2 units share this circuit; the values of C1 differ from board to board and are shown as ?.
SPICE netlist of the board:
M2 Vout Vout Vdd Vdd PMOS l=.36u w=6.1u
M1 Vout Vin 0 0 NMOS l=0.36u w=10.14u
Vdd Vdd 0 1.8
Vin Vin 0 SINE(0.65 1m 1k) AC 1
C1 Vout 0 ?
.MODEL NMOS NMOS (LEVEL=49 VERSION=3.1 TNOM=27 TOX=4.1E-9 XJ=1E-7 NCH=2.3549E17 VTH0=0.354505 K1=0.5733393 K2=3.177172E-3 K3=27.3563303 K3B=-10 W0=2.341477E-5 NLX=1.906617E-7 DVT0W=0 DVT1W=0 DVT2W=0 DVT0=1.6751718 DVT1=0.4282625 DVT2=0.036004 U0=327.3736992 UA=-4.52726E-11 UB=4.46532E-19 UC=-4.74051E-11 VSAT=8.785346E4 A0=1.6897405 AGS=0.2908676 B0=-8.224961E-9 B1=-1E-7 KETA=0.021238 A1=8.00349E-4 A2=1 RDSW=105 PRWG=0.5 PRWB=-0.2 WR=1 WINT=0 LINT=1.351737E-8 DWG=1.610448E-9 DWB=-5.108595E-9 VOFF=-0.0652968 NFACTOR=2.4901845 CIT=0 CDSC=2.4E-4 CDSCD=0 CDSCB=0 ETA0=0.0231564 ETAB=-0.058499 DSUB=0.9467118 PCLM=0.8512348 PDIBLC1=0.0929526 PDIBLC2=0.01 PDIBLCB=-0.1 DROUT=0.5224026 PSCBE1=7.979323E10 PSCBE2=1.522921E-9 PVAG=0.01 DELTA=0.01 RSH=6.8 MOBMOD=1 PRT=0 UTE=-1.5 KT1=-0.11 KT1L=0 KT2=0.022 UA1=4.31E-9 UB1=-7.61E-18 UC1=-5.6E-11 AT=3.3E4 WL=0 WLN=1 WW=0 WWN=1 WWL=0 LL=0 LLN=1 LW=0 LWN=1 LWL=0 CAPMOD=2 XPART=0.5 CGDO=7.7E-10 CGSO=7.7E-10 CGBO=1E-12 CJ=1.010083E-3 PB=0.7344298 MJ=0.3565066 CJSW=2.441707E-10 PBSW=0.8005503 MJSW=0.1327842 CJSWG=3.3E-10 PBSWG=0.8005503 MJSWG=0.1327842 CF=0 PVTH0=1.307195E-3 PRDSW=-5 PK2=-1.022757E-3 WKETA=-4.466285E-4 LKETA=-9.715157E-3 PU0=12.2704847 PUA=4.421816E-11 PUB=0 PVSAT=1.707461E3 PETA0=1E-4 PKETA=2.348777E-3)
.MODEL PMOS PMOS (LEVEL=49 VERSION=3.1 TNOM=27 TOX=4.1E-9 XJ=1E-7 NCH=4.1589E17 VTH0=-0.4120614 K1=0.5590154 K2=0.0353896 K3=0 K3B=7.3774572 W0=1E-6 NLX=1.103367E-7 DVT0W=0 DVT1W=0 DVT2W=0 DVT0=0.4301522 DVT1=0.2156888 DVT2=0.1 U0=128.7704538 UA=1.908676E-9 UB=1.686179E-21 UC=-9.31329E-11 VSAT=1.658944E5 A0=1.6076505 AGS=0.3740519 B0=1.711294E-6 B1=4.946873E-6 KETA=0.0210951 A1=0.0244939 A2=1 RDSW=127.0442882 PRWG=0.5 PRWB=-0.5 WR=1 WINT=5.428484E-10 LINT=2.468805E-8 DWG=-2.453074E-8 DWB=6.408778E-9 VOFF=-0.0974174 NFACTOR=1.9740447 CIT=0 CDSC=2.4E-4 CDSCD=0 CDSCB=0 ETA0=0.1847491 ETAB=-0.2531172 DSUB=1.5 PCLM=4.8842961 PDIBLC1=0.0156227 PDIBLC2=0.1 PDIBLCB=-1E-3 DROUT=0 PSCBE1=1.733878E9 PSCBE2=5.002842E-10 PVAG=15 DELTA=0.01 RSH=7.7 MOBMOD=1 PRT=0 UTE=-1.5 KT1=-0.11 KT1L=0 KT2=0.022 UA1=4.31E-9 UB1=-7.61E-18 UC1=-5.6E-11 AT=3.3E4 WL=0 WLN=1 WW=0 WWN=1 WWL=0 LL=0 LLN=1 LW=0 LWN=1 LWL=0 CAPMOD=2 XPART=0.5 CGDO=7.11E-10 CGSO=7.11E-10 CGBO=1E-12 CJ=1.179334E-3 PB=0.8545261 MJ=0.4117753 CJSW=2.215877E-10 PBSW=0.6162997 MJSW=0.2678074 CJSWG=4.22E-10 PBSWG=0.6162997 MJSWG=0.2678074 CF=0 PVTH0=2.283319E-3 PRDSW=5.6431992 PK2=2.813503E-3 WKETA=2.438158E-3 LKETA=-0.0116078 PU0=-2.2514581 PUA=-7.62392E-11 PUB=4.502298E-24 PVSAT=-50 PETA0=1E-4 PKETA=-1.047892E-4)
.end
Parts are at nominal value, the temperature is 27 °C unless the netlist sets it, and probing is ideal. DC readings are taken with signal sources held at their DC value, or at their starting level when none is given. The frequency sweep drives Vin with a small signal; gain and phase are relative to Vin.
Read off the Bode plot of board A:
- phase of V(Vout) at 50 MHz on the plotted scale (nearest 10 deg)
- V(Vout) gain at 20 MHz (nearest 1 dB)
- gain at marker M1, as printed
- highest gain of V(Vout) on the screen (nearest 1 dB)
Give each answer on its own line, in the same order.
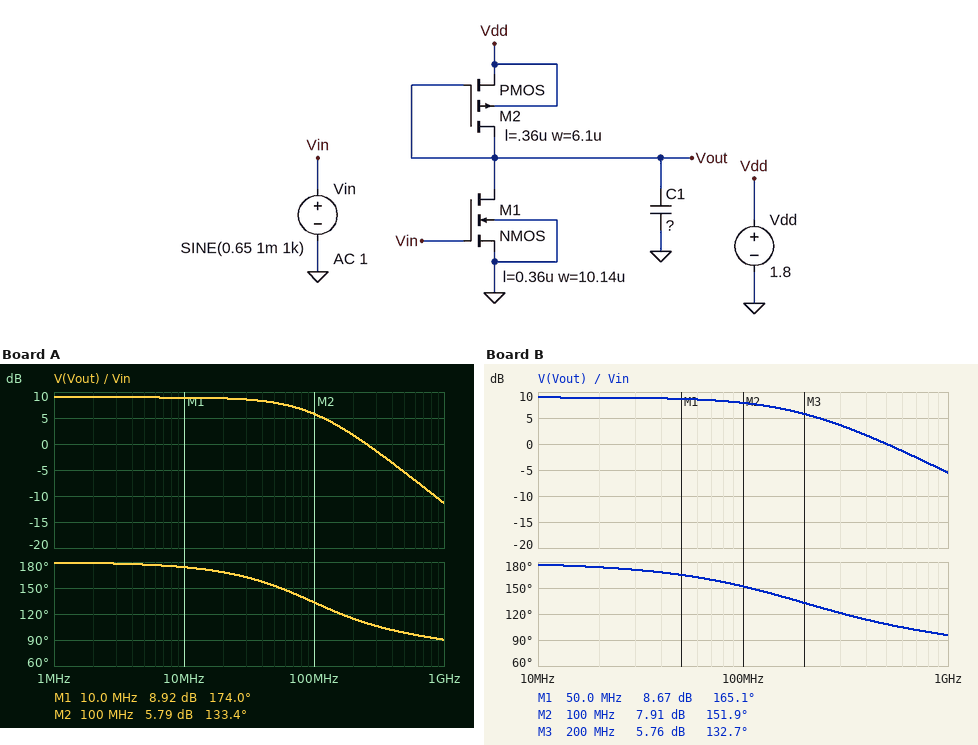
150 deg
9 dB
8.92 dB
9 dB
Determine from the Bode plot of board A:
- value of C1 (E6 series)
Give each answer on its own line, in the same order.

680 fF
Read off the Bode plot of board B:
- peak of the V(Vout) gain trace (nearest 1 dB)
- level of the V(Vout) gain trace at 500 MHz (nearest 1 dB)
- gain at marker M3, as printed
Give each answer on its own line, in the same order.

9 dB
0 dB
5.76 dB
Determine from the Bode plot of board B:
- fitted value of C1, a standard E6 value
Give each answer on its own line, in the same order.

330 fF
